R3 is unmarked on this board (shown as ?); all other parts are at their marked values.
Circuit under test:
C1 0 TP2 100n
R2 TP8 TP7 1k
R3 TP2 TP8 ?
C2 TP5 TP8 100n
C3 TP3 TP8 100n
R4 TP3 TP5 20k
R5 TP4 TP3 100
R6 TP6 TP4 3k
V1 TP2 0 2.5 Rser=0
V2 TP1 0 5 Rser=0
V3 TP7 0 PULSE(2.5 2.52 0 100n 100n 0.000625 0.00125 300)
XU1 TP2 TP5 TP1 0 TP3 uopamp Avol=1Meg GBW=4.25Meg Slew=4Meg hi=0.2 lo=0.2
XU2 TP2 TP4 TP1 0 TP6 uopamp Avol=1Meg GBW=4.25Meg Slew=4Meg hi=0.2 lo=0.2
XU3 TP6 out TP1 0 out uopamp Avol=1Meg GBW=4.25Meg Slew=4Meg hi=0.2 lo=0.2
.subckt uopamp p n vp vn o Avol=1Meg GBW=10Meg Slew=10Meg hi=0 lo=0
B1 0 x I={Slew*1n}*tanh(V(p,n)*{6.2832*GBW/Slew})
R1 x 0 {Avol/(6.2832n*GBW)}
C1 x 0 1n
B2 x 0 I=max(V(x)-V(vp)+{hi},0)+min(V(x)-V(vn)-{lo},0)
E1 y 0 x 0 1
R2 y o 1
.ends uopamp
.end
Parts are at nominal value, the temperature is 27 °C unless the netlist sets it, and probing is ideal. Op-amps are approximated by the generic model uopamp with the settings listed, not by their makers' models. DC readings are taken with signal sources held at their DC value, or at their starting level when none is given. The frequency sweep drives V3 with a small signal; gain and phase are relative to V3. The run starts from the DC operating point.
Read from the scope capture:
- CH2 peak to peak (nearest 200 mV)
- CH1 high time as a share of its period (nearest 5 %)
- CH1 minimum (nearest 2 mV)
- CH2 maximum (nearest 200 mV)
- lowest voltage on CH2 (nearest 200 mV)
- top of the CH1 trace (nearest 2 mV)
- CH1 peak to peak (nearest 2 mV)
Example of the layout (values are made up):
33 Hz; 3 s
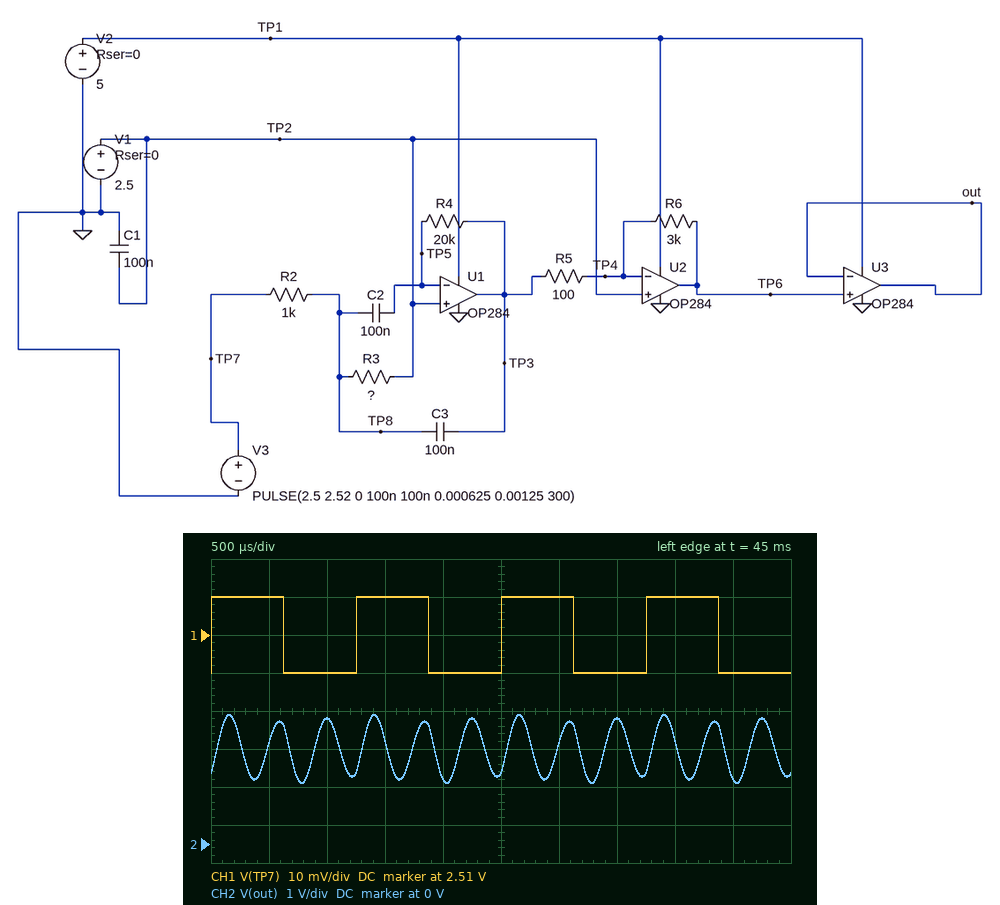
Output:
1.8 V; 50 %; 2.500 V; 3.4 V; 1.6 V; 2.520 V; 20 mV
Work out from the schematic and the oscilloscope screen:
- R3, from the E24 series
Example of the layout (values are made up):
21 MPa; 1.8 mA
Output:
24 Ω
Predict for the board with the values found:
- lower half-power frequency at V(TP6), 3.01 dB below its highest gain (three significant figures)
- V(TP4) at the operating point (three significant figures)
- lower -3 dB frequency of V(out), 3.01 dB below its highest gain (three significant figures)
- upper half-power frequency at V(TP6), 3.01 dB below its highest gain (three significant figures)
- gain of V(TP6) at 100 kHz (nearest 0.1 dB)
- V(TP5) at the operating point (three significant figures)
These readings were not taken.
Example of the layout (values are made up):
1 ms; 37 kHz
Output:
2.23 kHz; 2.50 V; 2.23 kHz; 2.39 kHz; -8.4 dB; 2.50 V
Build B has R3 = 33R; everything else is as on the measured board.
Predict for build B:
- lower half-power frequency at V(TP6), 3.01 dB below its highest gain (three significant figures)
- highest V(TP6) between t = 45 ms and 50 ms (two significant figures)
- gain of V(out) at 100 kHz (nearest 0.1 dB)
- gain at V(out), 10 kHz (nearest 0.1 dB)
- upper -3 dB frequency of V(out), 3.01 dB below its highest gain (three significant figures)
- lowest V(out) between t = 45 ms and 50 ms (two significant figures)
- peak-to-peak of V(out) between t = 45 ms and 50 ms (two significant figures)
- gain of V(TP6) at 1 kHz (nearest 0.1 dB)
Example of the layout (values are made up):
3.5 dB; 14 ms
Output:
1.90 kHz; 2.8 V; -8.4 dB; 13.8 dB; 2.06 kHz; 2.2 V; 680 mV; 24.2 dB
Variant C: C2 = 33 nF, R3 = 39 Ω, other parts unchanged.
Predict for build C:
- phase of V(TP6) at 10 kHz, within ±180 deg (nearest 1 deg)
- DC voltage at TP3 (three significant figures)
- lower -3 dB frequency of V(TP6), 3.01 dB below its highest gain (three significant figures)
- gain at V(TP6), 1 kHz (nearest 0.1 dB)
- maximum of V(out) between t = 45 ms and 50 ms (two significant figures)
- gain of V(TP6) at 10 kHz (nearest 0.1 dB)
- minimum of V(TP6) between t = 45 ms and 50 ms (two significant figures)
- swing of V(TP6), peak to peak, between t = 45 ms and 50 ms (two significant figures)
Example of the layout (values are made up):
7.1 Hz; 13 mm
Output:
-92 deg; 2.50 V; 3.03 kHz; 14.3 dB; 2.7 V; 14.4 dB; 2.3 V; 360 mV
